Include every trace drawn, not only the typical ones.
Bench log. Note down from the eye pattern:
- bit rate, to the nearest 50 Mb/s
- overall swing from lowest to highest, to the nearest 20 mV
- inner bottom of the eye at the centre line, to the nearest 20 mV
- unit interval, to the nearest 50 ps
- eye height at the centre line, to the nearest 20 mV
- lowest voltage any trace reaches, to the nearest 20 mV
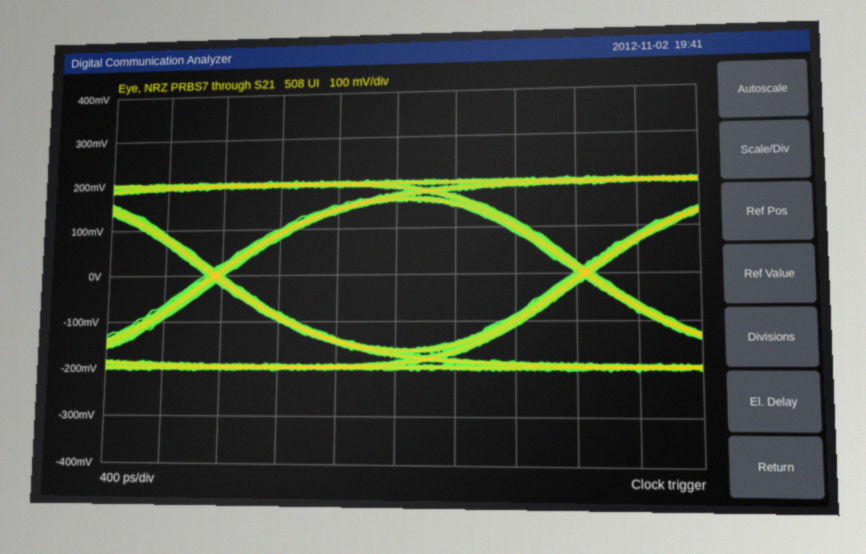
400 Mb/s
420 mV
-160 mV
2.50 ns
320 mV
-200 mV
